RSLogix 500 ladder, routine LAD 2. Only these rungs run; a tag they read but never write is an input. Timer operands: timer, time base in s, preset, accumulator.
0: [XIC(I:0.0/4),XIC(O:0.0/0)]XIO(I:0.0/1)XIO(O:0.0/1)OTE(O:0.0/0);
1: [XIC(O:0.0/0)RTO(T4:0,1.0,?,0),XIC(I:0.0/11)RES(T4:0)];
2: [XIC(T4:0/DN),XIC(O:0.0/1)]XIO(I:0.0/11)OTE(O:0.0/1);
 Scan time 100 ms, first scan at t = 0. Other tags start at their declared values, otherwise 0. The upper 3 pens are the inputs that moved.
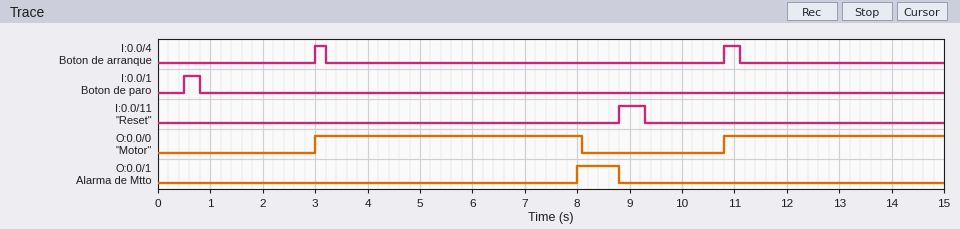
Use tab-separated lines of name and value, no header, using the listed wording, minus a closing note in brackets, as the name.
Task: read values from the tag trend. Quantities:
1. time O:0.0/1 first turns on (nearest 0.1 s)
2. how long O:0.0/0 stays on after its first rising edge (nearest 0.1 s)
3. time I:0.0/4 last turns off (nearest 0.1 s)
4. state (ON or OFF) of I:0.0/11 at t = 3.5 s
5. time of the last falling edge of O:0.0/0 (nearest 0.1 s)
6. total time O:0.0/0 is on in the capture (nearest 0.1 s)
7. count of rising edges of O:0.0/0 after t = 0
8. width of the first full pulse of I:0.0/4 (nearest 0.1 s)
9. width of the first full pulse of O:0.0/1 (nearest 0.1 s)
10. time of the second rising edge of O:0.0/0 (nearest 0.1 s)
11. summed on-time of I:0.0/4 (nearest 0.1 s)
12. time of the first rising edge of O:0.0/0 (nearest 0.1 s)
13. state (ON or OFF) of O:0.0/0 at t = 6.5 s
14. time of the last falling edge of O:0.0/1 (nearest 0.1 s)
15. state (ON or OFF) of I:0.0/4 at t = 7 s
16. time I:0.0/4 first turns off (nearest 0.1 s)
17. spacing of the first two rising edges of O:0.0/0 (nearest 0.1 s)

time O:0.0/1 first turns on	8.0 s
how long O:0.0/0 stays on after its first rising edge	5.1 s
time I:0.0/4 last turns off	11.1 s
state (ON or OFF) of I:0.0/11 at t = 3.5 s	OFF
time of the last falling edge of O:0.0/0	8.1 s
total time O:0.0/0 is on in the capture	9.3 s
count of rising edges of O:0.0/0 after t = 0	2
width of the first full pulse of I:0.0/4	0.2 s
width of the first full pulse of O:0.0/1	0.8 s
time of the second rising edge of O:0.0/0	10.8 s
summed on-time of I:0.0/4	0.5 s
time of the first rising edge of O:0.0/0	3.0 s
state (ON or OFF) of O:0.0/0 at t = 6.5 s	ON
time of the last falling edge of O:0.0/1	8.8 s
state (ON or OFF) of I:0.0/4 at t = 7 s	OFF
time I:0.0/4 first turns off	3.2 s
spacing of the first two rising edges of O:0.0/0	7.8 s
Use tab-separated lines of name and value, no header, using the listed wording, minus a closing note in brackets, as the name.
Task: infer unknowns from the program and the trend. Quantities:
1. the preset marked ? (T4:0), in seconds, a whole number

the preset marked ? (T4:0), in seconds, a whole number	5 s
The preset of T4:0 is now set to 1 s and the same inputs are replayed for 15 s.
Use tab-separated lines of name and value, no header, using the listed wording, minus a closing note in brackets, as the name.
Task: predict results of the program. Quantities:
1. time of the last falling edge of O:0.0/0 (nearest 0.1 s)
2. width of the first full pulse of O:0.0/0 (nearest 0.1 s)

time of the last falling edge of O:0.0/0	11.9 s
width of the first full pulse of O:0.0/0	1.1 s
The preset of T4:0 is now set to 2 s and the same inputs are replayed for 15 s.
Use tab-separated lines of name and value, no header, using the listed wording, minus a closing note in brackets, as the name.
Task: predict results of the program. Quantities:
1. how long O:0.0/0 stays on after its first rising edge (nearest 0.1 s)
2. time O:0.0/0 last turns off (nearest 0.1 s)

how long O:0.0/0 stays on after its first rising edge	2.1 s
time O:0.0/0 last turns off	12.9 s
